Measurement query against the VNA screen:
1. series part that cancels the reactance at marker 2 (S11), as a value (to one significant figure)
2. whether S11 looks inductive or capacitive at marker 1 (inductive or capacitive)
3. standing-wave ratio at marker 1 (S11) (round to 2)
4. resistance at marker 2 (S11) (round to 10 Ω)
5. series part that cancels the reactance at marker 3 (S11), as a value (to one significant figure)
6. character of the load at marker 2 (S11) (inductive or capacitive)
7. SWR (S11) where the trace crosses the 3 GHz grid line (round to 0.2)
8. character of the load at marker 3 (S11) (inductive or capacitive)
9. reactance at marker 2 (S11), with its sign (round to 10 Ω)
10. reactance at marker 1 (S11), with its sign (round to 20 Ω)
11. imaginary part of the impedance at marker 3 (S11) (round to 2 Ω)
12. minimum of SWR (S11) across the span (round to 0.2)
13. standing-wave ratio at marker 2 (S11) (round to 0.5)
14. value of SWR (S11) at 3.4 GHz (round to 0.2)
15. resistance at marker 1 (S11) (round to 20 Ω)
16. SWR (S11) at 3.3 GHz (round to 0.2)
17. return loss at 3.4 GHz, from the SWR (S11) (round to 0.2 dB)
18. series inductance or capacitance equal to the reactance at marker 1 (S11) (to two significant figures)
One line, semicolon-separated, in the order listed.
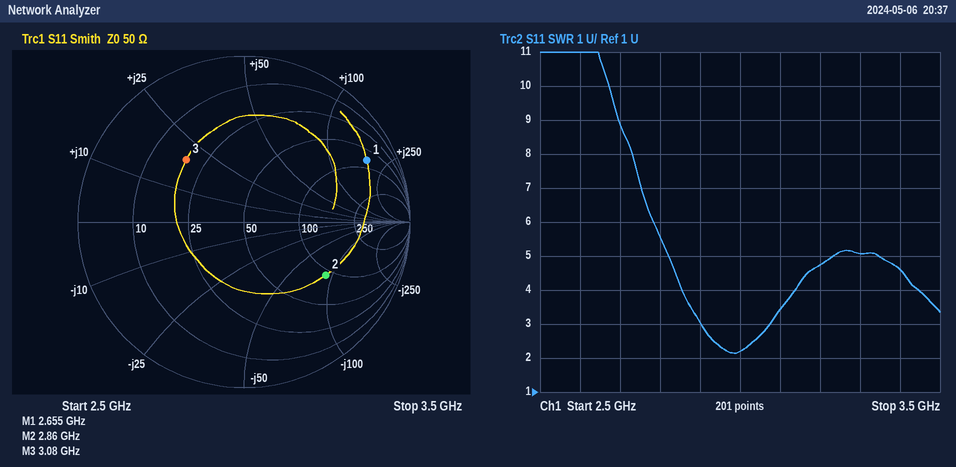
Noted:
5 nH; inductive; 10; 90 Ω; 3 pF; capacitive; 2.2; inductive; -90 Ω; +180 Ω; +20 Ω; 2.2; 4.0; 4.6; 80 Ω; 5.0; 3.8 dB; 11 nH
